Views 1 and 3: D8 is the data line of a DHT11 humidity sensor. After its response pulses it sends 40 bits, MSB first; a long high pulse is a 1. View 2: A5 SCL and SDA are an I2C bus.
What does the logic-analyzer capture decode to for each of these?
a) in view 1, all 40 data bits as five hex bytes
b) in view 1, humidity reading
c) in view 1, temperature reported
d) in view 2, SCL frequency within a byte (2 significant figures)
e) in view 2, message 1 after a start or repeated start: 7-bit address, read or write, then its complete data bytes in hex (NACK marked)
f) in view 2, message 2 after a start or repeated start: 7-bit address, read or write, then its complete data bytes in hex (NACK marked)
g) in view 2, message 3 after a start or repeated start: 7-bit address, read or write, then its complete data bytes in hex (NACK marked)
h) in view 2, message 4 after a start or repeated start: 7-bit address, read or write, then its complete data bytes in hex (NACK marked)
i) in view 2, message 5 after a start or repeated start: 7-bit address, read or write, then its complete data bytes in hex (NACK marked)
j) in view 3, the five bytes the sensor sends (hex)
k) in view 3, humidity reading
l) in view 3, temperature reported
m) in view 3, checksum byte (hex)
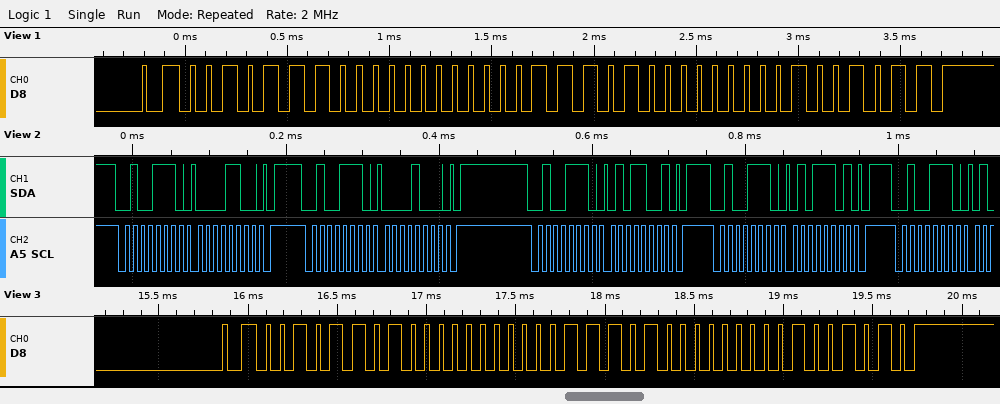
2E 00 1D 00 4B
46 %
29.0 °C
100 kHz
0x27 write: 0C
0x27 write: 08
0x27 write: 59
0x27 write: 5D
0x27 write
2D 00 1D 00 4A
45 %
29.0 °C
0x4A
